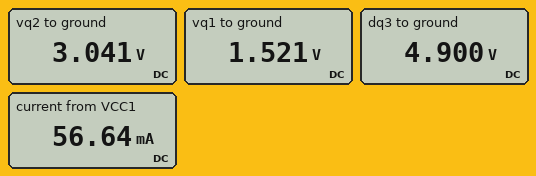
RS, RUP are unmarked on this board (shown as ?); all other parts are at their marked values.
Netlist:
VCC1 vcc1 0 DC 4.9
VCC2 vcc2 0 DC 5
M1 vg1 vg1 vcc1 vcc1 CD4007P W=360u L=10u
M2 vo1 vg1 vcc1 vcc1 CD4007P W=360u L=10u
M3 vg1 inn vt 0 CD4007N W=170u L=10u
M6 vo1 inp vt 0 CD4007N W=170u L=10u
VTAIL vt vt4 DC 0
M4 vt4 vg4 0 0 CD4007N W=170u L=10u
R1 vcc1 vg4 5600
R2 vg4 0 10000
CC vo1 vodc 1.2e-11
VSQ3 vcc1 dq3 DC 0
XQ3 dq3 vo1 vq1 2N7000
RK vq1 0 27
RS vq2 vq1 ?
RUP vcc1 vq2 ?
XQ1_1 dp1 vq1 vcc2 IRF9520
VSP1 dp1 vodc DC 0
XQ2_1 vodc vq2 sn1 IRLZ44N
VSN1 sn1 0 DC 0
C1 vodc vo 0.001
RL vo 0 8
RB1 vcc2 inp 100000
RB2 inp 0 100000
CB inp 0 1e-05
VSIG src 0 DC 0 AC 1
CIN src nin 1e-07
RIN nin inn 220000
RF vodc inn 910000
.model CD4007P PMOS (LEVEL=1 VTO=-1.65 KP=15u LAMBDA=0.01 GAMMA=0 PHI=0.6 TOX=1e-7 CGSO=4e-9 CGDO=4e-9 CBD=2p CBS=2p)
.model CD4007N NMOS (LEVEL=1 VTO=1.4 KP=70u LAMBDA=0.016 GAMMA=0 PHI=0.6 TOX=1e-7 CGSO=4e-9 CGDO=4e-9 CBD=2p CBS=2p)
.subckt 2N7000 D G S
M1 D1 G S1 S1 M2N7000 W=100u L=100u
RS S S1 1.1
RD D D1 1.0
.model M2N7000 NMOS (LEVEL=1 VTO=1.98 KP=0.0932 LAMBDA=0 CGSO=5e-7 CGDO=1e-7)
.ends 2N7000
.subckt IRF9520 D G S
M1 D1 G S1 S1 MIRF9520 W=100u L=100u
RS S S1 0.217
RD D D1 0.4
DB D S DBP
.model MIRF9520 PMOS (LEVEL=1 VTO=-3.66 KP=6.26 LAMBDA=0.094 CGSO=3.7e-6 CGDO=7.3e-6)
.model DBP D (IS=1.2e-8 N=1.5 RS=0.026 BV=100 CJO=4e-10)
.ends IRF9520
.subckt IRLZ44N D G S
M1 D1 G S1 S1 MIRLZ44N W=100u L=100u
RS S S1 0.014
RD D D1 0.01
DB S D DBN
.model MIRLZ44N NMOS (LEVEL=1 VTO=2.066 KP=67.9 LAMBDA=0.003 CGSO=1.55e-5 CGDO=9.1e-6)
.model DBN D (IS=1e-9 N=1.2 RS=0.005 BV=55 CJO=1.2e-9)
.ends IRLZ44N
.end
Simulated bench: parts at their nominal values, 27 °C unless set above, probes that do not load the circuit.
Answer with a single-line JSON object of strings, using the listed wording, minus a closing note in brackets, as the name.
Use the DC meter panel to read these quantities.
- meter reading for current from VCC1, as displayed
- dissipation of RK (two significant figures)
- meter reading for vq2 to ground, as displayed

{"meter reading for current from VCC1, as displayed": "56.64 mA", "dissipation of RK": "86 mW", "meter reading for vq2 to ground, as displayed": "3.041 V"}
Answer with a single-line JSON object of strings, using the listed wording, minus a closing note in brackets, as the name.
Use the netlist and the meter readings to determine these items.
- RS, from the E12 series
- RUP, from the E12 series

{"RS, from the E12 series": "27 Ω", "RUP, from the E12 series": "33 Ω"}
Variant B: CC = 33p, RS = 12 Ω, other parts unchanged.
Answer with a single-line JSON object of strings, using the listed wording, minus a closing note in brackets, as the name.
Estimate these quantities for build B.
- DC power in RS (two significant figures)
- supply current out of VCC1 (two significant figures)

{"DC power in RS": "56 mW", "supply current out of VCC1": "68 mA"}
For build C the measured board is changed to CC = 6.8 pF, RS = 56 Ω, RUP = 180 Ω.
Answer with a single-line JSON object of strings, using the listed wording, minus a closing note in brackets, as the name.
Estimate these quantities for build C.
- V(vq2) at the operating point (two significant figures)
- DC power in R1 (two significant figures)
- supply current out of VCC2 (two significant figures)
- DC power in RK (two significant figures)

{"V(vq2) at the operating point": "2.1 V", "DC power in R1": "550 µW", "supply current out of VCC2": "40 mA", "DC power in RK": "56 mW"}
